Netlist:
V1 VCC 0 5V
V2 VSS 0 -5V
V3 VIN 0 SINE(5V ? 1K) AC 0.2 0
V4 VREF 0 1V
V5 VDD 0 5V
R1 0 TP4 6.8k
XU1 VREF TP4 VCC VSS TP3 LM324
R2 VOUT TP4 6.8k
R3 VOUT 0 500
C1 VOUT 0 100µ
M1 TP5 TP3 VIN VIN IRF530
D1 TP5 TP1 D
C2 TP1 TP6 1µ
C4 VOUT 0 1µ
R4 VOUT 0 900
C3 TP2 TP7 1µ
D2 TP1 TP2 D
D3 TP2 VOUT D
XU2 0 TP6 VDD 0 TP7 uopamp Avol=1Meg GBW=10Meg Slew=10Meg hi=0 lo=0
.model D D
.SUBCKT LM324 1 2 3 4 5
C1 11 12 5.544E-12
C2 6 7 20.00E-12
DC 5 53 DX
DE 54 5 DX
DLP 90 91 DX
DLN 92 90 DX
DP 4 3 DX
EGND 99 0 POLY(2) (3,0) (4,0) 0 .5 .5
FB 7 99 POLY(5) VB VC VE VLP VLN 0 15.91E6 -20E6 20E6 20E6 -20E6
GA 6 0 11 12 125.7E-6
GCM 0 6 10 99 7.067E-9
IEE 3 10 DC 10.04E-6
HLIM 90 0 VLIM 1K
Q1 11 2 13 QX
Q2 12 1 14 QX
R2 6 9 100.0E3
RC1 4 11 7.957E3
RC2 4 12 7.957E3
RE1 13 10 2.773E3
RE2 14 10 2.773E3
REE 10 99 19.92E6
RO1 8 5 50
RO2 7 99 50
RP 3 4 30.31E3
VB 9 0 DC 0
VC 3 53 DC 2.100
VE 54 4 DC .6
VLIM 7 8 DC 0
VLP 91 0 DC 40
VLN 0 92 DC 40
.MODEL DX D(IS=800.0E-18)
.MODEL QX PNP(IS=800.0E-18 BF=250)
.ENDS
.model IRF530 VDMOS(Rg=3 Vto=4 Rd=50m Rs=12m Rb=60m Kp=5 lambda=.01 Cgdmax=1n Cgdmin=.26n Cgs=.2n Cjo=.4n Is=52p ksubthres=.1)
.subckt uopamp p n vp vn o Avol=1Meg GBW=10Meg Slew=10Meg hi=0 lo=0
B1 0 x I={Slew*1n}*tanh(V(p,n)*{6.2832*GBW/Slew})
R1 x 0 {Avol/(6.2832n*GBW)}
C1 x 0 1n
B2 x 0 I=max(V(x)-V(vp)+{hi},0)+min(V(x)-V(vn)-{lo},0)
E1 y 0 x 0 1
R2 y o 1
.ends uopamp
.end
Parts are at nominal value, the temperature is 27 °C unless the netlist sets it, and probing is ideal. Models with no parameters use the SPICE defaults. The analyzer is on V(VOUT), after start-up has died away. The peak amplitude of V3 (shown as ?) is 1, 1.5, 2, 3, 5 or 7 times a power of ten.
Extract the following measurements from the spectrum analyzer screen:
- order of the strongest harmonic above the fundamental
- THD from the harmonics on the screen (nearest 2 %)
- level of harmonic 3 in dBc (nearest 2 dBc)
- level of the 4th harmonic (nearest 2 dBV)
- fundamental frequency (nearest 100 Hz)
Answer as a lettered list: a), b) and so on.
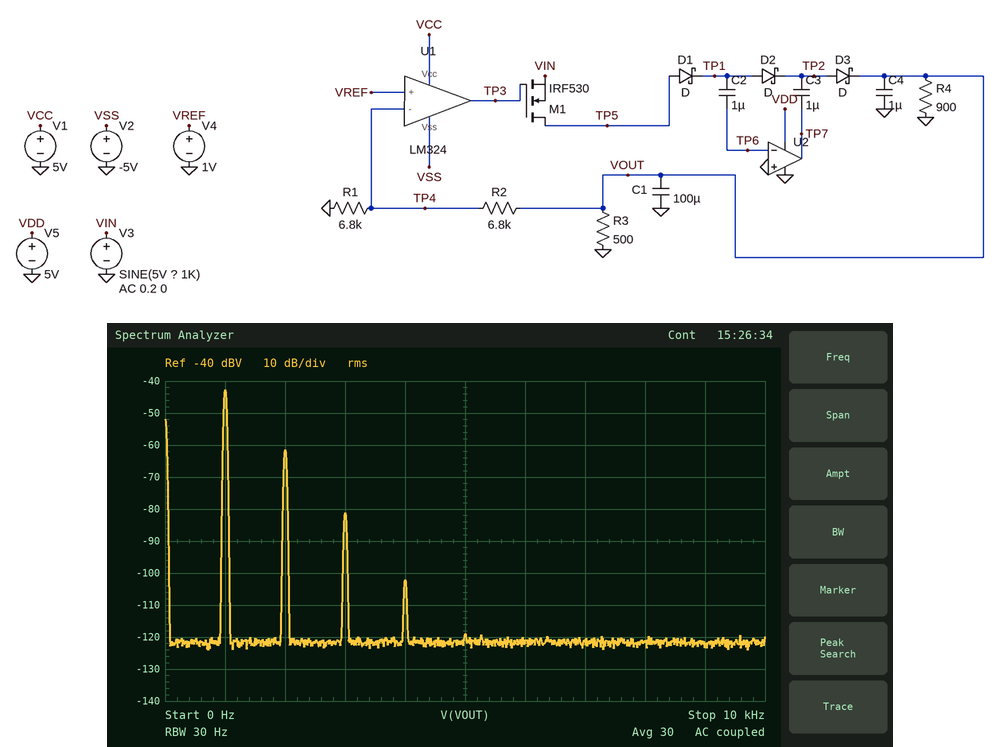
a) 2
b) 12 %
c) -38 dBc
d) -102 dBV
e) 1.0 kHz
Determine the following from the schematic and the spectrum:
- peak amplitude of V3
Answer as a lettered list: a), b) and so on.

a) 100 mV
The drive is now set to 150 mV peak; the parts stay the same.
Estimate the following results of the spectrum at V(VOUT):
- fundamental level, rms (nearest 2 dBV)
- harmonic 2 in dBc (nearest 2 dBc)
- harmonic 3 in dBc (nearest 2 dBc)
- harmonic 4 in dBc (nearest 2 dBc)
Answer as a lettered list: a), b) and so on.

a) -40 dBV
b) -16 dBc
c) -32 dBc
d) -50 dBc
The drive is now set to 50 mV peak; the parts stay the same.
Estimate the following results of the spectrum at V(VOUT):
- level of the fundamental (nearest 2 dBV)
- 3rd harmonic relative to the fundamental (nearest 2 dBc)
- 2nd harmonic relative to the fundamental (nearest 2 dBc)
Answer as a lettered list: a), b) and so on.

a) -48 dBV
b) -50 dBc
c) -24 dBc
